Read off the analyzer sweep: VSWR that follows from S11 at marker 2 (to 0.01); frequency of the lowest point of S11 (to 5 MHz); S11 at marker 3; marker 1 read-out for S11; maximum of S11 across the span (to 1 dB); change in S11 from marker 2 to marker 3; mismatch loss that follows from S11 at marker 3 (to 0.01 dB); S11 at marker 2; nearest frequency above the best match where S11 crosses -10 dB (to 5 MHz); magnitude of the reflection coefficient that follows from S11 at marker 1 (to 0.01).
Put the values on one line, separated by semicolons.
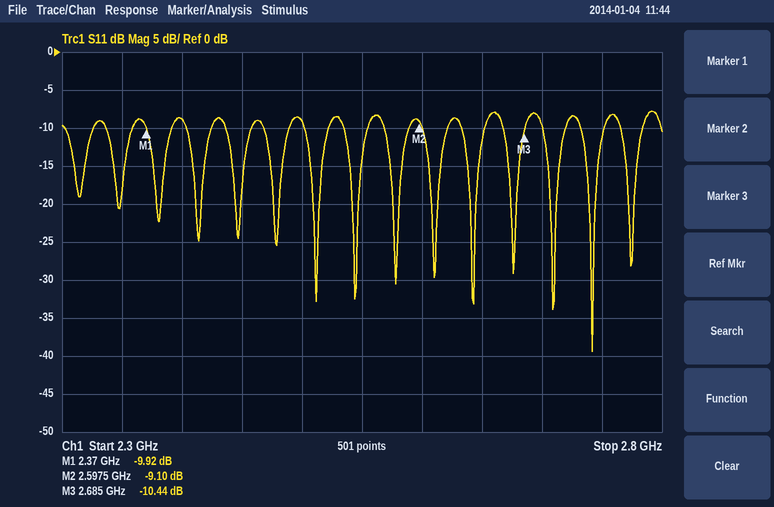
2.08; 2.740 GHz; -10.44 dB; -9.92 dB; -8 dB; -1.34 dB; 0.41 dB; -9.10 dB; 2.750 GHz; 0.32
